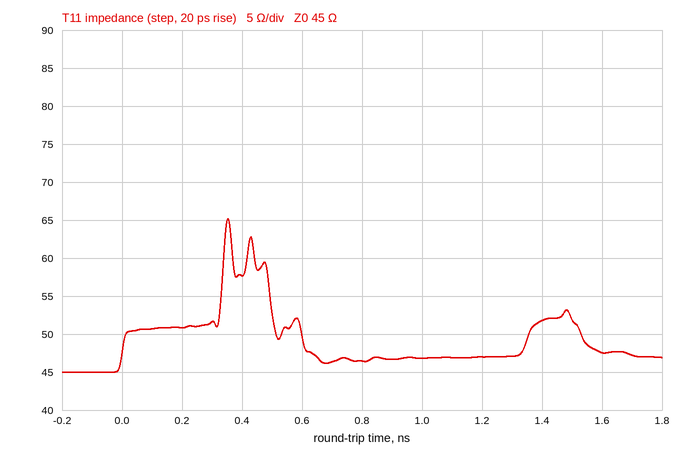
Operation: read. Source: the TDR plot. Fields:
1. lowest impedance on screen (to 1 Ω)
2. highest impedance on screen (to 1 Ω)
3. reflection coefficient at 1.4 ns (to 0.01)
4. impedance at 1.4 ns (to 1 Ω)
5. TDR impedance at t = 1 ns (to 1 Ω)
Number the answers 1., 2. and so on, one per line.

1. 45 Ω
2. 65 Ω
3. +0.07
4. 52 Ω
5. 47 Ω
